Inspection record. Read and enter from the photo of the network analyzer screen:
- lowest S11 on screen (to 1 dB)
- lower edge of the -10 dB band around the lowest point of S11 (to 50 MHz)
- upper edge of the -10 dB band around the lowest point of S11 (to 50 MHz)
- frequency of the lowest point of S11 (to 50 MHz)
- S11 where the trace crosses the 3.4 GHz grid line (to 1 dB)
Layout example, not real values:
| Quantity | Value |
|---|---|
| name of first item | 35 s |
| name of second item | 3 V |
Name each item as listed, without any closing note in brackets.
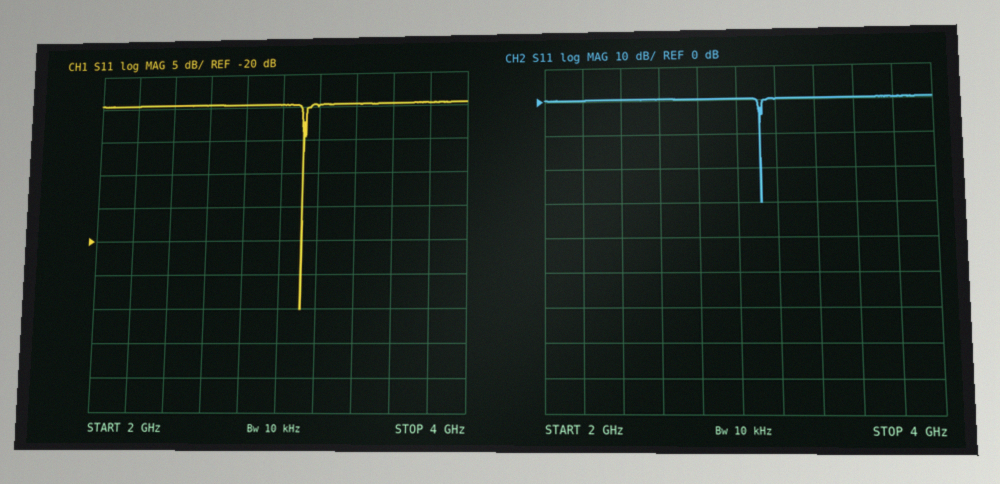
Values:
| Quantity | Value |
|---|---|
| lowest S11 on screen | -30 dB |
| lower edge of the -10 dB band around the lowest point of S11 | 3.10 GHz |
| upper edge of the -10 dB band around the lowest point of S11 | 3.10 GHz |
| frequency of the lowest point of S11 | 3.10 GHz |
| S11 where the trace crosses the 3.4 GHz grid line | 0 dB |
